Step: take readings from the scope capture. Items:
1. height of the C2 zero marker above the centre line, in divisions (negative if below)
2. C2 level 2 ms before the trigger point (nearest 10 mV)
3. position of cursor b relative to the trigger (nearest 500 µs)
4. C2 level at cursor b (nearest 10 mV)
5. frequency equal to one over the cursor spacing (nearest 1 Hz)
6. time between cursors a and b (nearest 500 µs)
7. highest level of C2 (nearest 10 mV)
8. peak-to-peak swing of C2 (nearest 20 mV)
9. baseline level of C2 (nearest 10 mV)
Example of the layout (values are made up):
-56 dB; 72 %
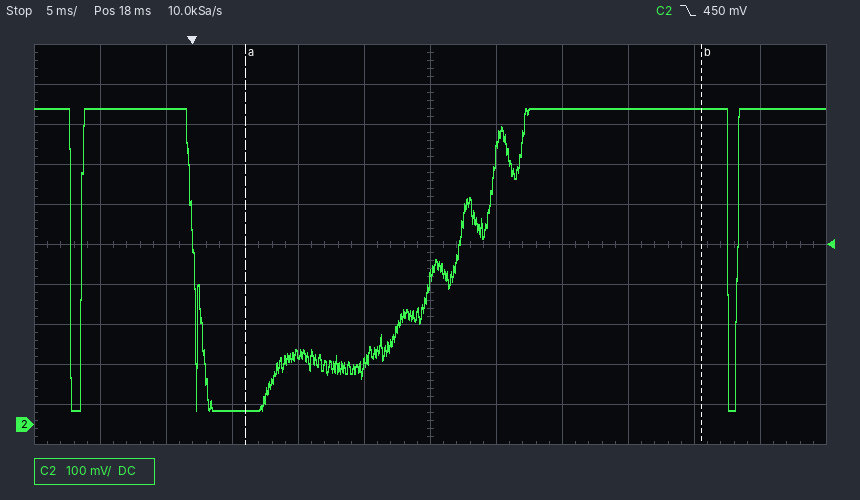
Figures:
-4.5 div; 790 mV; +38.5 ms; 790 mV; 29 Hz; 34.5 ms; 790 mV; 760 mV; 790 mV
